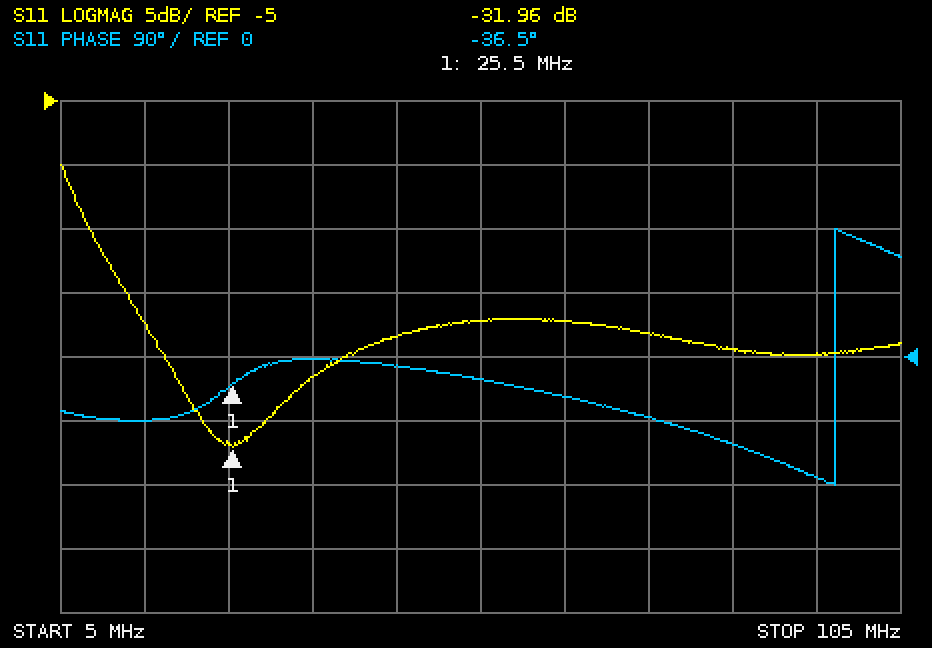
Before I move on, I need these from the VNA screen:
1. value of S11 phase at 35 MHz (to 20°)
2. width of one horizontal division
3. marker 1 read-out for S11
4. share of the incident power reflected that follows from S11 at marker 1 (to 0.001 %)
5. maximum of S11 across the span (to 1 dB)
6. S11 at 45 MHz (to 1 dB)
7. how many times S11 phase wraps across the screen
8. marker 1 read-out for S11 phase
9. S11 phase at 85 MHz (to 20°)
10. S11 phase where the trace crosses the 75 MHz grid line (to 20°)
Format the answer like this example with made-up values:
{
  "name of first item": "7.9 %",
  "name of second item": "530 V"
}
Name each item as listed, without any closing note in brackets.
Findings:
{
  "value of S11 phase at 35 MHz": "0°",
  "width of one horizontal division": "10 MHz",
  "marker 1 read-out for S11": "-31.96 dB",
  "share of the incident power reflected that follows from S11 at marker 1": "0.064 %",
  "maximum of S11 across the span": "-10 dB",
  "S11 at 45 MHz": "-23 dB",
  "how many times S11 phase wraps across the screen": "1",
  "marker 1 read-out for S11 phase": "-36.5°",
  "S11 phase at 85 MHz": "-120°",
  "S11 phase where the trace crosses the 75 MHz grid line": "-80°"
}
